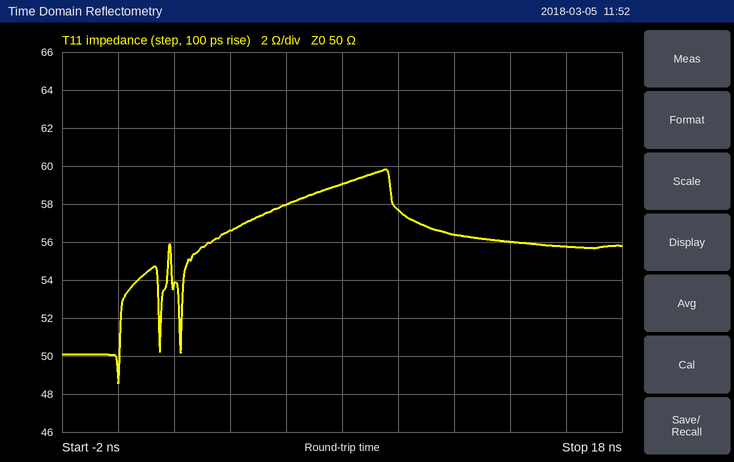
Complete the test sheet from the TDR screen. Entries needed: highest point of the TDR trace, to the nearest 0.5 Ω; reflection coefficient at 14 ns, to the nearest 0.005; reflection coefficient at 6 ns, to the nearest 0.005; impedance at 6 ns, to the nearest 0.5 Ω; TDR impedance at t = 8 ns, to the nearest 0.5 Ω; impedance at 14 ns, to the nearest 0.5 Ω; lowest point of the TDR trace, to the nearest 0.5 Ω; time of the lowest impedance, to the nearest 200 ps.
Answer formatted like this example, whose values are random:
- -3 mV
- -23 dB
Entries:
- 60.0 Ω
- +0.055
- +0.075
- 58.0 Ω
- 59.0 Ω
- 56.0 Ω
- 48.5 Ω
- 0.0 ns
